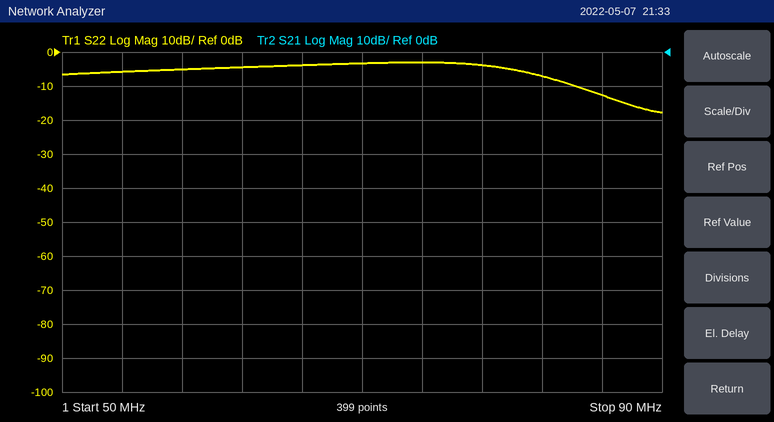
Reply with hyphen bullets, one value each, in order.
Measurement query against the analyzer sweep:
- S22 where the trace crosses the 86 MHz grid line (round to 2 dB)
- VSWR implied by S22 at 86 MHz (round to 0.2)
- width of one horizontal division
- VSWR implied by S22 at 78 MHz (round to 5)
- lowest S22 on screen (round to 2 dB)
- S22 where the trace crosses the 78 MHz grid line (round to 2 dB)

- -12 dB
- 1.6
- 4 MHz
- 5
- -18 dB
- -4 dB
